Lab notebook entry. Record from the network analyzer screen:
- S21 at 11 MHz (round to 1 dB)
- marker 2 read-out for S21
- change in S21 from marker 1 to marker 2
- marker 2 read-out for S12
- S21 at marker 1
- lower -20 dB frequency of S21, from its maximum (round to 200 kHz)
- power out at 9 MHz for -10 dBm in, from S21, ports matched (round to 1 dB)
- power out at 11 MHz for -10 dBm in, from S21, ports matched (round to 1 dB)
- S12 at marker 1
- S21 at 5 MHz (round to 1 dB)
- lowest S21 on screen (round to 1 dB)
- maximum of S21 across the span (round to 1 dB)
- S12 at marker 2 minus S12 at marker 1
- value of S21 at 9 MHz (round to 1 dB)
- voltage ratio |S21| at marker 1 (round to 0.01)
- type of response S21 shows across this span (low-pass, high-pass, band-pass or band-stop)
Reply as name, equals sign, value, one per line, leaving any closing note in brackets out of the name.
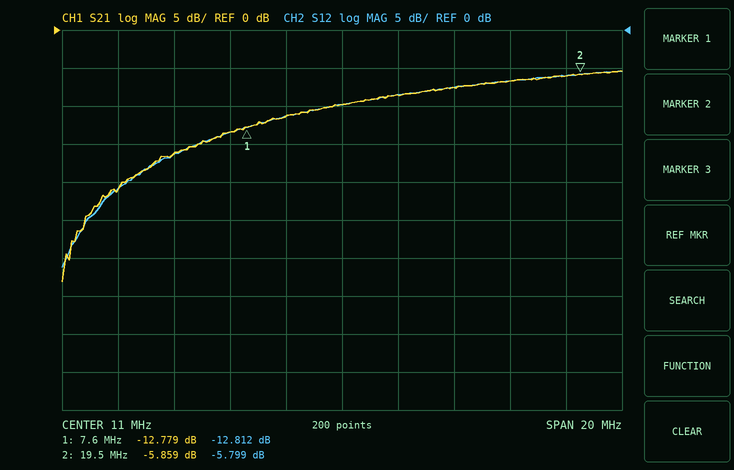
S21 at 11 MHz = -10 dB
marker 2 read-out for S21 = -5.859 dB
change in S21 from marker 1 to marker 2 = 6.920 dB
marker 2 read-out for S12 = -5.799 dB
S21 at marker 1 = -12.779 dB
lower -20 dB frequency of S21, from its maximum = 1.8 MHz
power out at 9 MHz for -10 dBm in, from S21, ports matched = -21 dBm
power out at 11 MHz for -10 dBm in, from S21, ports matched = -20 dBm
S12 at marker 1 = -12.812 dB
S21 at 5 MHz = -16 dB
lowest S21 on screen = -33 dB
maximum of S21 across the span = -5 dB
S12 at marker 2 minus S12 at marker 1 = 7.013 dB
value of S21 at 9 MHz = -11 dB
voltage ratio |S21| at marker 1 = 0.23
type of response S21 shows across this span = high-pass
